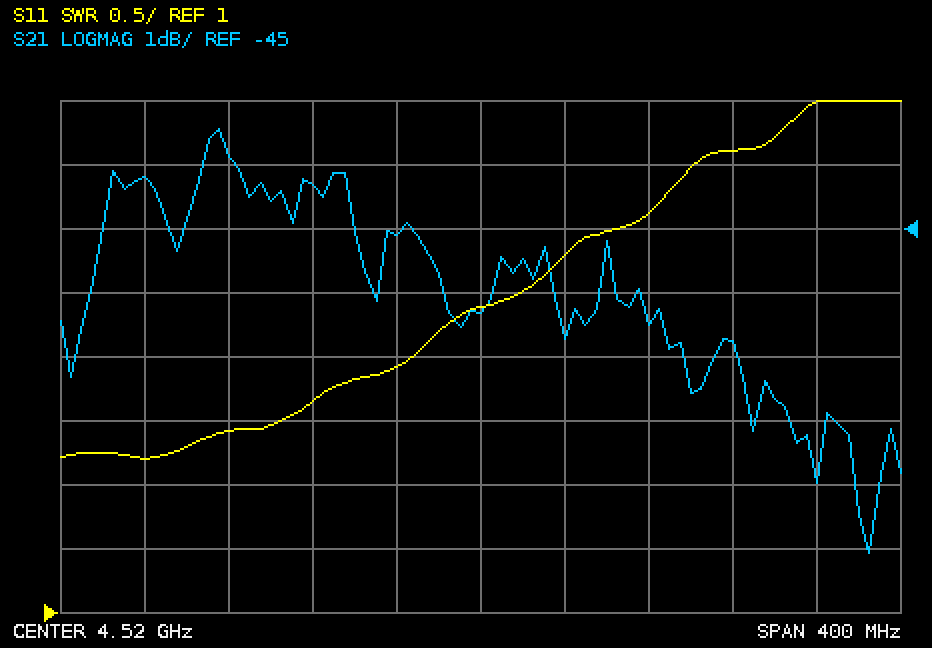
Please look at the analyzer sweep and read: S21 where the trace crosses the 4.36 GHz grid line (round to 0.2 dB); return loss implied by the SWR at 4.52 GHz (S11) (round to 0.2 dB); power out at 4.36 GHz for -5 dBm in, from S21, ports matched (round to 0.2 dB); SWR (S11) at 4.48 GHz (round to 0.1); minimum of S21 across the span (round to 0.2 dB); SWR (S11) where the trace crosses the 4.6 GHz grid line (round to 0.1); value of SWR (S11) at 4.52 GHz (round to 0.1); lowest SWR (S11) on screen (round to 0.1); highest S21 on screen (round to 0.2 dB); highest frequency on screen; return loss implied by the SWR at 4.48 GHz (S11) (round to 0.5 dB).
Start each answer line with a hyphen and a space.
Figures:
- -44.2 dB
- 5.2 dB
- -49.2 dBm
- 2.9
- -50.0 dB
- 4.1
- 3.4
- 2.2
- -43.4 dB
- 4.72 GHz
- 6.0 dB
